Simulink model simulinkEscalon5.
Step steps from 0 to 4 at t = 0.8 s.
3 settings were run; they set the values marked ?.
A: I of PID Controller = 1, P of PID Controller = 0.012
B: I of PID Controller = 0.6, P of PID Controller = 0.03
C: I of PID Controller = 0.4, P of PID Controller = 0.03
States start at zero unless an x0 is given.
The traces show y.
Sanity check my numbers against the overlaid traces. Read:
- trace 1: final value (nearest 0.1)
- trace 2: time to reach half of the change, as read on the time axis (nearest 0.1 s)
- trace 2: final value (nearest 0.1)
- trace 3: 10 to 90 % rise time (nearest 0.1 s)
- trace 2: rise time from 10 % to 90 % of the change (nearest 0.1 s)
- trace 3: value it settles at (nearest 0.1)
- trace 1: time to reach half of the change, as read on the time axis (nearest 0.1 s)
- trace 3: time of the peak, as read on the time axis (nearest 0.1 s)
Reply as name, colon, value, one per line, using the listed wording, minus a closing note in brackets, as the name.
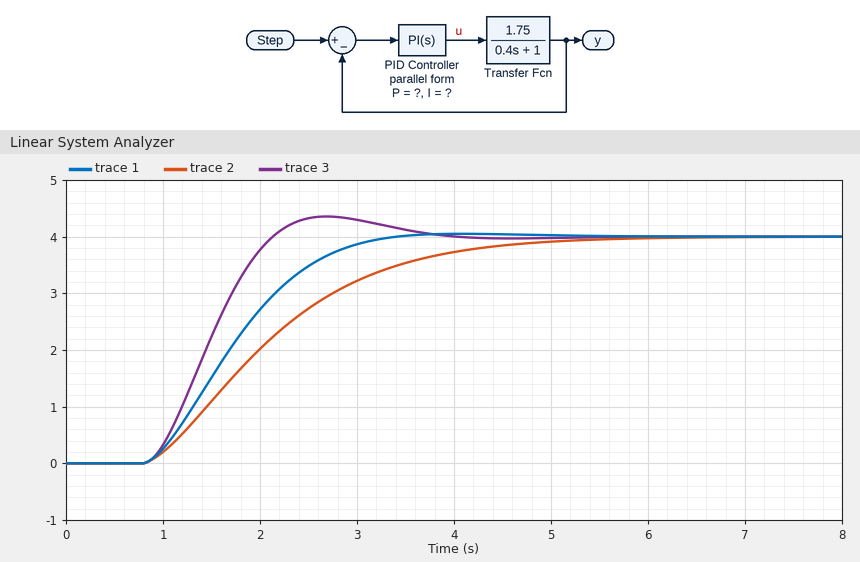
trace 1: final value: 4.0
trace 2: time to reach half of the change, as read on the time axis: 2.0 s
trace 2: final value: 4.0
trace 3: 10 to 90 % rise time: 0.9 s
trace 2: rise time from 10 % to 90 % of the change: 2.5 s
trace 3: value it settles at: 4.0
trace 1: time to reach half of the change, as read on the time axis: 1.7 s
trace 3: time of the peak, as read on the time axis: 2.7 s
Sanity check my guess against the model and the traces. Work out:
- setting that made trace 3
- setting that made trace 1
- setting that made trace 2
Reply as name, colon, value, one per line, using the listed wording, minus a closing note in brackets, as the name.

setting that made trace 3: A
setting that made trace 1: B
setting that made trace 2: C
